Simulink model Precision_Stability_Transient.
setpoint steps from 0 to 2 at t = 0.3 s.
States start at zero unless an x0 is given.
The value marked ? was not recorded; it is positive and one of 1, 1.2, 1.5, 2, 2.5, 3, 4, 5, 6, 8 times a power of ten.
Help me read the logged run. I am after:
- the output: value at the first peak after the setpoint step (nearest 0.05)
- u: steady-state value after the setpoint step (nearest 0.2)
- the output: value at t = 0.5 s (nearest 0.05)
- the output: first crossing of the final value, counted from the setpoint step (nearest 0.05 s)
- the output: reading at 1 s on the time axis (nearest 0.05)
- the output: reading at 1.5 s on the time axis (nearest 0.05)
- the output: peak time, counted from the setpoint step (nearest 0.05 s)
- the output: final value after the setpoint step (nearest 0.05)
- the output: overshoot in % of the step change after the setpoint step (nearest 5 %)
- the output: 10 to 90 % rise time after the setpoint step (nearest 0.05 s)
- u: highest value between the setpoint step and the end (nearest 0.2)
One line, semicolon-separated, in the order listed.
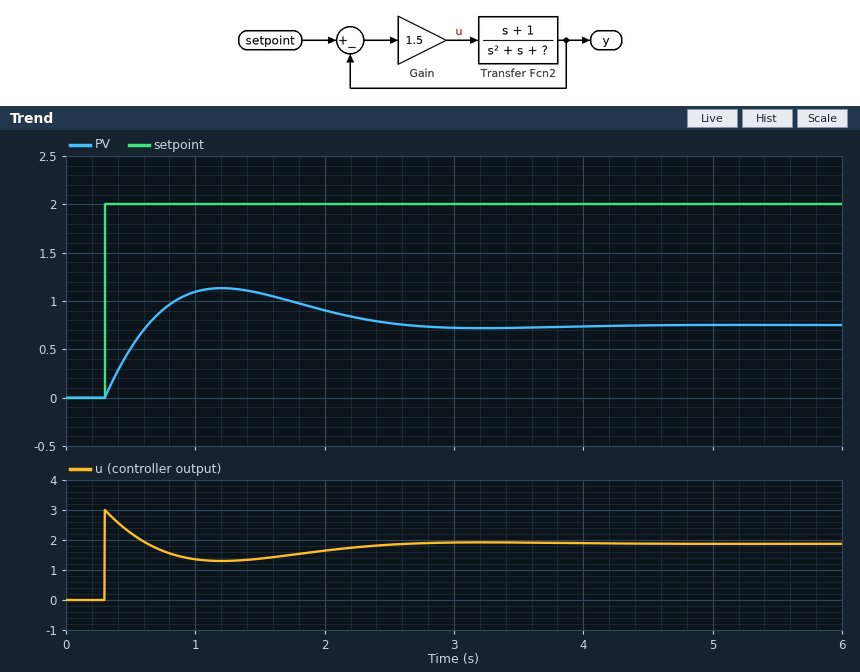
1.15; 1.8; 0.50; 0.35 s; 1.10; 1.10; 0.90 s; 0.75; 50 %; 0.25 s; 3.0
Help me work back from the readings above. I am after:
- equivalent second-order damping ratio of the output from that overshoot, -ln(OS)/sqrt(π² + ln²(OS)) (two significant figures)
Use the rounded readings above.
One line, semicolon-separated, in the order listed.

0.22
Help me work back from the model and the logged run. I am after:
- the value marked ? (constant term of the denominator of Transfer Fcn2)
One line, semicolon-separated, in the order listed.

2.5
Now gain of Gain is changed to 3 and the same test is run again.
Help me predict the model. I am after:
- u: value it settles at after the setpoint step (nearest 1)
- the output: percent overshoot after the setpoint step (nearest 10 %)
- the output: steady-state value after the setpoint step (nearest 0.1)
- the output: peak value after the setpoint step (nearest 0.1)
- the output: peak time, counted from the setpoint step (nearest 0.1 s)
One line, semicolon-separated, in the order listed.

3; 40 %; 1.1; 1.5; 0.7 s
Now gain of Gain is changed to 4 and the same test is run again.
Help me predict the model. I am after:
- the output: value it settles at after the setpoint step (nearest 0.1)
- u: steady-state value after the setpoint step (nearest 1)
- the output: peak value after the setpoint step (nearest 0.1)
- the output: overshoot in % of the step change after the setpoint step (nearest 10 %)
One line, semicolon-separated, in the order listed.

1.2; 3; 1.6; 30 %
